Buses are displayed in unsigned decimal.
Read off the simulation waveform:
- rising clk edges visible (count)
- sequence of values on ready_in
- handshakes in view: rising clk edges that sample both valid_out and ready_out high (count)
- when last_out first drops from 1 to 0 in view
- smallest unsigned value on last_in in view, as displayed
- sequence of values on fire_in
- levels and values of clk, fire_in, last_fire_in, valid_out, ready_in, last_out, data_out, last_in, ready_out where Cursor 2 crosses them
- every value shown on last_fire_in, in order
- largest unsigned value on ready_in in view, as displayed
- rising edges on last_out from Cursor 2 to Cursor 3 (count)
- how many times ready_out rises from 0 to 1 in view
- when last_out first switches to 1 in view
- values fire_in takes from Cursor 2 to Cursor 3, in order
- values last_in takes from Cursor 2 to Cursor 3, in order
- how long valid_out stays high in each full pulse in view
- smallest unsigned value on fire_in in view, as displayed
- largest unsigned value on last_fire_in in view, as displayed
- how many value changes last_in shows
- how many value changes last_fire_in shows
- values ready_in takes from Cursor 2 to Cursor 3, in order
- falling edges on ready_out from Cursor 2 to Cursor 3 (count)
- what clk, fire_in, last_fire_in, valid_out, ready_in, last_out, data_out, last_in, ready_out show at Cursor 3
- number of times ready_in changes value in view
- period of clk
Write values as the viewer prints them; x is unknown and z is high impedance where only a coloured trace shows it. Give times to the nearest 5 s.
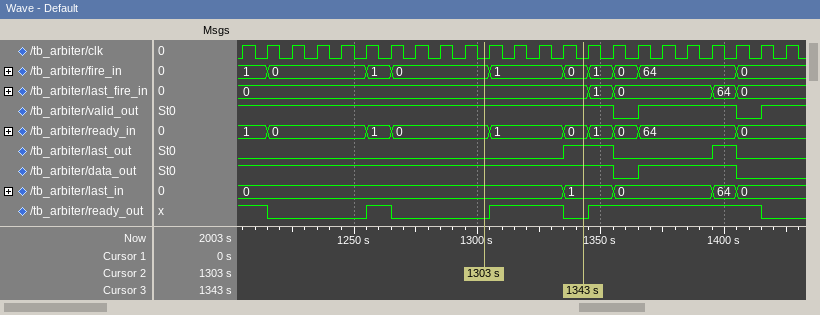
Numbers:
23
1, 0, 1, 0, 1, 0, 1, 0, 64, 0
11
1355 s
0
1, 0, 1, 0, 1, 0, 1, 0, 64, 0
clk=0, fire_in=0, last_fire_in=0, valid_out=1, ready_in=0, last_out=0, data_out=1, last_in=0, ready_out=0
0, 1, 0, 64, 0
64
1
3
1335 s
0, 1, 0
0, 1
40 s
0
64
4
4
0, 1, 0
1
clk=0, fire_in=0, last_fire_in=0, valid_out=1, ready_in=0, last_out=1, data_out=1, last_in=1, ready_out=0
9
10 s
